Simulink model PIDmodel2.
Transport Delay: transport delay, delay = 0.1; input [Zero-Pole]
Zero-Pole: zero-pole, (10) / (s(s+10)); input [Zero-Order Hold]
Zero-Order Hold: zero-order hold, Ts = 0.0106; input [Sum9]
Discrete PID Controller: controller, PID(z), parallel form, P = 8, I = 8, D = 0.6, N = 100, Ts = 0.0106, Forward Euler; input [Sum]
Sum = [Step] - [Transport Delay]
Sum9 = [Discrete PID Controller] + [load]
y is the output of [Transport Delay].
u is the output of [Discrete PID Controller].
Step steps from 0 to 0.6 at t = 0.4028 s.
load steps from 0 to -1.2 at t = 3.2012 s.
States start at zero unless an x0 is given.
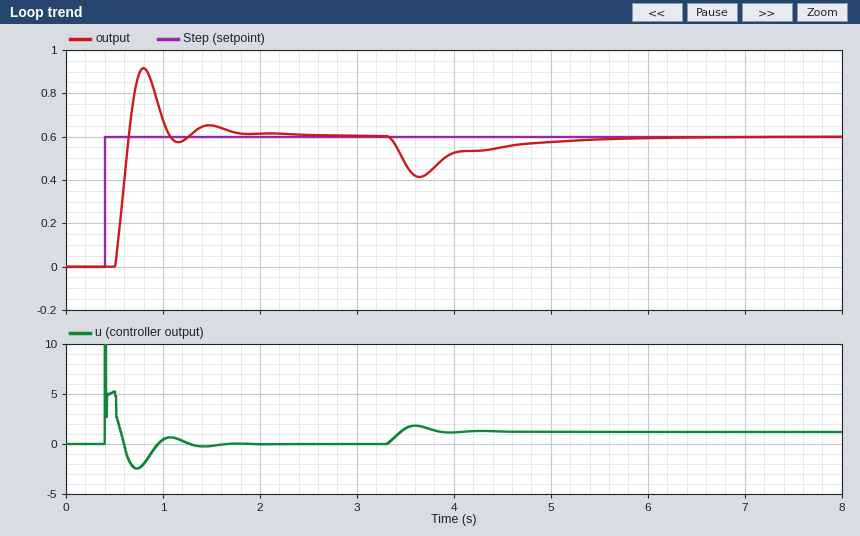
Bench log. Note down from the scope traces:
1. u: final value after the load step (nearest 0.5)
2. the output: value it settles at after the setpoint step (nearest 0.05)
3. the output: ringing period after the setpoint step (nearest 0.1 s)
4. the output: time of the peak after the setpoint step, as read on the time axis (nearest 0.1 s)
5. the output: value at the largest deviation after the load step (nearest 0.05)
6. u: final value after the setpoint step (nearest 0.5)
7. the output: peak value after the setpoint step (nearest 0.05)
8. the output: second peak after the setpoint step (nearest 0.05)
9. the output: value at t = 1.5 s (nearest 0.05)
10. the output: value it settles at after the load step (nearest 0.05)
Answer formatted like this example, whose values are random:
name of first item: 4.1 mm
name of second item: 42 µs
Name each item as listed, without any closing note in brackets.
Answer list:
u: final value after the load step: 1.0
the output: value it settles at after the setpoint step: 0.60
the output: ringing period after the setpoint step: 0.7 s
the output: time of the peak after the setpoint step, as read on the time axis: 0.8 s
the output: value at the largest deviation after the load step: 0.40
u: final value after the setpoint step: 0.0
the output: peak value after the setpoint step: 0.90
the output: second peak after the setpoint step: 0.65
the output: value at t = 1.5 s: 0.65
the output: value it settles at after the load step: 0.60
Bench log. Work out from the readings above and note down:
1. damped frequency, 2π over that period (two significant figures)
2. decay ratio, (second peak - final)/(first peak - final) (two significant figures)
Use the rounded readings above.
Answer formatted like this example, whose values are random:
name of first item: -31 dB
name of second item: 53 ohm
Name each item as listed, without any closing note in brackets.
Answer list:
damped frequency, 2π over that period: 9.0 rad/s
decay ratio, (second peak - final)/(first peak - final): 0.17
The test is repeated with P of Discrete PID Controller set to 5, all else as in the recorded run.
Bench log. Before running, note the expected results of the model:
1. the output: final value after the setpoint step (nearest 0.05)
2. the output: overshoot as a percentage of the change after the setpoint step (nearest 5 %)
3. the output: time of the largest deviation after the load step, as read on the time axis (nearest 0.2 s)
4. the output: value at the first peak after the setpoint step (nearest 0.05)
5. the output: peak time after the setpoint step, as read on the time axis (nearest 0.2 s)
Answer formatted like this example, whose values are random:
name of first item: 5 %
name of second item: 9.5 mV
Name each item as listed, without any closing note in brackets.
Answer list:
the output: final value after the setpoint step: 0.60
the output: overshoot as a percentage of the change after the setpoint step: 25 %
the output: time of the largest deviation after the load step, as read on the time axis: 3.8 s
the output: value at the first peak after the setpoint step: 0.75
the output: peak time after the setpoint step, as read on the time axis: 1.0 s
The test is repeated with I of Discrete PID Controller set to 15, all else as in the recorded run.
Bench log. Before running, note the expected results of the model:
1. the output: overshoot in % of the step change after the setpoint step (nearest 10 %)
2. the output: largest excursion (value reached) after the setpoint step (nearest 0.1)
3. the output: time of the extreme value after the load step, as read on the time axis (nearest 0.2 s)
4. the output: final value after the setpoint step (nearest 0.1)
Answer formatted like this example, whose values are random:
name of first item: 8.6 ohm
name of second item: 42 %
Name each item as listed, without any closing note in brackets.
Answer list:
the output: overshoot in % of the step change after the setpoint step: 70 %
the output: largest excursion (value reached) after the setpoint step: 1.0
the output: time of the extreme value after the load step, as read on the time axis: 3.6 s
the output: final value after the setpoint step: 0.6
